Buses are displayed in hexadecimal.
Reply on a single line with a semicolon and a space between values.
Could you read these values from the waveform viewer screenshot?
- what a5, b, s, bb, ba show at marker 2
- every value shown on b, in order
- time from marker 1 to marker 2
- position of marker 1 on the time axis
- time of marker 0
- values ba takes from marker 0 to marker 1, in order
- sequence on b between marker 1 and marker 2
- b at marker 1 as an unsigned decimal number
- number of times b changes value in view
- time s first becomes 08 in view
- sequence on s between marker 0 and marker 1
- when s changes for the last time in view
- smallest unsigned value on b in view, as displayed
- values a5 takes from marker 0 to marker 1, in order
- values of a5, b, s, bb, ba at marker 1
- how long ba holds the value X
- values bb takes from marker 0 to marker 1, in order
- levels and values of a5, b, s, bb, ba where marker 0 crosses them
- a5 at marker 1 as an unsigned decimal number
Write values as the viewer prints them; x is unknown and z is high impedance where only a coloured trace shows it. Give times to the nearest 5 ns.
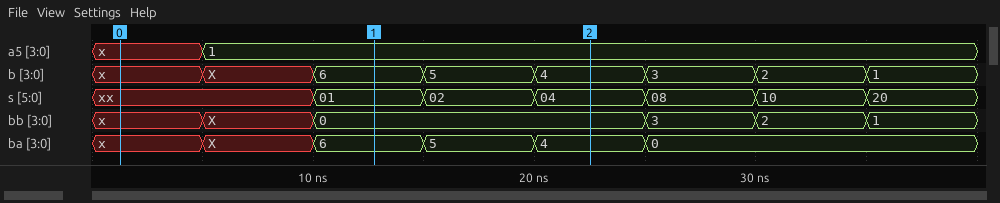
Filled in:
a5=1, b=4, s=04, bb=0, ba=4; x, X, 6, 5, 4, 3, 2, 1; 10 ns; 15 ns; 0 ns; x, X, 6; 6, 5, 4; 6; 7; 25 ns; xx, 01; 35 ns; 1; x, 1; a5=1, b=6, s=01, bb=0, ba=6; 5 ns; x, X, 0; a5=x, b=x, s=xx, bb=x, ba=x; 1
